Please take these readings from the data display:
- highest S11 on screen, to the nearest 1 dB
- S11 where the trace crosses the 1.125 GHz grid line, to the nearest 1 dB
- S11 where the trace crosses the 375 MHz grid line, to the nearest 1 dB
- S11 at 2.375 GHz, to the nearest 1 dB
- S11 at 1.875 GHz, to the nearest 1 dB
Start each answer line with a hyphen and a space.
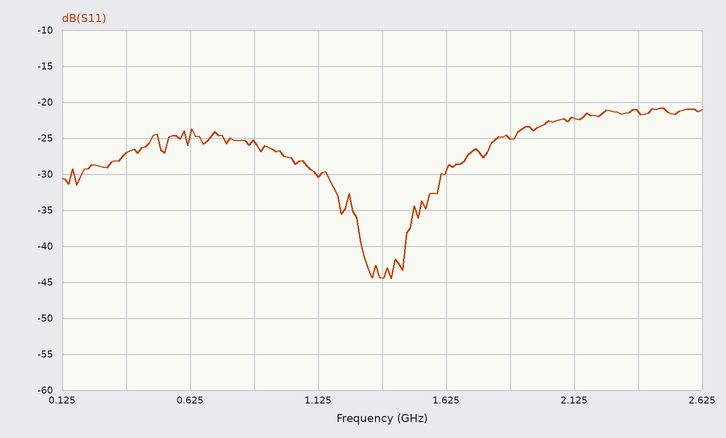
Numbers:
- -21 dB
- -30 dB
- -27 dB
- -21 dB
- -25 dB
